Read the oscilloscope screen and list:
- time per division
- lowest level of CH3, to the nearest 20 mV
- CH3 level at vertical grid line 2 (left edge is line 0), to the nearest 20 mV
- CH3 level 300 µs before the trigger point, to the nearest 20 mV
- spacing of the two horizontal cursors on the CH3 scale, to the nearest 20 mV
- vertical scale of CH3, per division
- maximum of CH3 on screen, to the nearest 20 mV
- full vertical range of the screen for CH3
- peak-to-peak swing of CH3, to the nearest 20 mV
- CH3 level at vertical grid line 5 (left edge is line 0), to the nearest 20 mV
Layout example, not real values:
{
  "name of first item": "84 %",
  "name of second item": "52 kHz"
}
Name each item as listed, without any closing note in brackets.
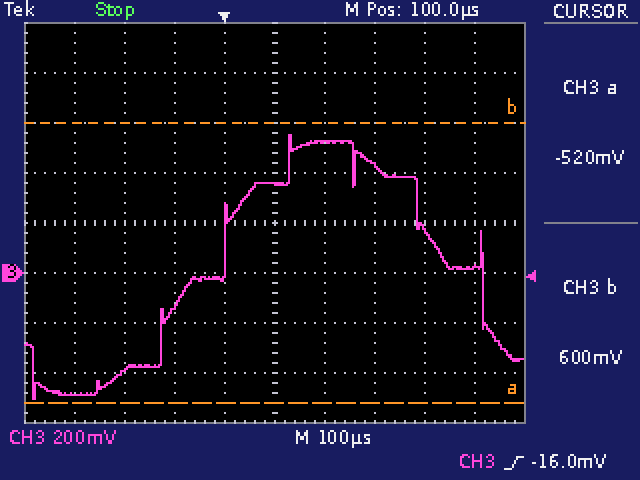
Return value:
{
  "time per division": "100 µs",
  "lowest level of CH3, to the nearest 20 mV": "-500 mV",
  "CH3 level at vertical grid line 2 (left edge is line 0), to the nearest 20 mV": "-400 mV",
  "CH3 level 300 µs before the trigger point, to the nearest 20 mV": "-480 mV",
  "spacing of the two horizontal cursors on the CH3 scale, to the nearest 20 mV": "1.12 V",
  "vertical scale of CH3, per division": "200 mV",
  "maximum of CH3 on screen, to the nearest 20 mV": "560 mV",
  "full vertical range of the screen for CH3": "1.6 V",
  "peak-to-peak swing of CH3, to the nearest 20 mV": "1.06 V",
  "CH3 level at vertical grid line 5 (left edge is line 0), to the nearest 20 mV": "360 mV"
}
